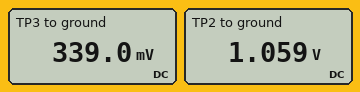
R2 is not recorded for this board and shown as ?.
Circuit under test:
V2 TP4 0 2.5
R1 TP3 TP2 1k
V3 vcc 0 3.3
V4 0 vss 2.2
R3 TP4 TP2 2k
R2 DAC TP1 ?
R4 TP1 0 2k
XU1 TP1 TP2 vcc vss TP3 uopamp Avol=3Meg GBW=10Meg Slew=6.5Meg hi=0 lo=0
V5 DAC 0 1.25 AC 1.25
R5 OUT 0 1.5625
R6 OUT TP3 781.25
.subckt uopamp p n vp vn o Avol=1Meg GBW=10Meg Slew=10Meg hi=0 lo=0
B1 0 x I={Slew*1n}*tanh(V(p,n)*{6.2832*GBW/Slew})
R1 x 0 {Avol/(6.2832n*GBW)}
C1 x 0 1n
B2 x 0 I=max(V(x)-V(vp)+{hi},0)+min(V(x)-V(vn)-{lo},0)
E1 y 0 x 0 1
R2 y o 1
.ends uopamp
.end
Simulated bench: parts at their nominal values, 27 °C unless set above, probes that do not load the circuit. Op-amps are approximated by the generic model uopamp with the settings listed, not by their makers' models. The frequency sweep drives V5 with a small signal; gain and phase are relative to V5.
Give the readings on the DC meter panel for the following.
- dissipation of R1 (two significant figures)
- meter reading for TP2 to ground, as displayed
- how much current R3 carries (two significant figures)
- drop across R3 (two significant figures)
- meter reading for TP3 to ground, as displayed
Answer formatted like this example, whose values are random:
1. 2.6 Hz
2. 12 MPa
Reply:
1. 520 µW
2. 1.059 V
3. 720 µA
4. 1.4 V
5. 339.0 mV
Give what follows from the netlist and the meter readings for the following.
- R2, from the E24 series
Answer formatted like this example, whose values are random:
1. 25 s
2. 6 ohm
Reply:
1. 360 Ω
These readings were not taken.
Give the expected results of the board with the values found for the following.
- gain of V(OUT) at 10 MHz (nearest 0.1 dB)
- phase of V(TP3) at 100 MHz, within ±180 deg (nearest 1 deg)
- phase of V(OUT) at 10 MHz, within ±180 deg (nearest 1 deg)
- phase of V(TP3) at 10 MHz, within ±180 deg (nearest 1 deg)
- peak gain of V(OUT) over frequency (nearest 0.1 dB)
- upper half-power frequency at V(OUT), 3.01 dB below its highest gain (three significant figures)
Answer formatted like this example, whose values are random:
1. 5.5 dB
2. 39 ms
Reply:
1. -57.0 dB
2. -86 deg
3. -56 deg
4. -56 deg
5. -51.9 dB
6. 6.66 MHz
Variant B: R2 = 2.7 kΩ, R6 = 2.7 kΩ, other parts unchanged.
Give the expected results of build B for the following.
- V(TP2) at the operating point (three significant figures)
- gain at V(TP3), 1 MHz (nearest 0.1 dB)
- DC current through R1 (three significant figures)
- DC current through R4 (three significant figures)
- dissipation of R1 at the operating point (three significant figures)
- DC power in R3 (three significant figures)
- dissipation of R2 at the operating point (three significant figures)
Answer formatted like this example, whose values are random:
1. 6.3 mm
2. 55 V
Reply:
1. 532 mV
2. -4.0 dB
3. 984 µA
4. 266 µA
5. 968 µW
6. 1.94 mW
7. 191 µW
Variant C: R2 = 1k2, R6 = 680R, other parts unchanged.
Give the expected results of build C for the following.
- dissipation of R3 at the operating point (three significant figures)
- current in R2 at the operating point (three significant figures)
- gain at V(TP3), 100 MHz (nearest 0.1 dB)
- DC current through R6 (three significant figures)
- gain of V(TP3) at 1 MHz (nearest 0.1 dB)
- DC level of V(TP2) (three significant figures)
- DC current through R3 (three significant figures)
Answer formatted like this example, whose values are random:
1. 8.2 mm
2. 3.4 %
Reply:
1. 1.48 mW
2. 391 µA
3. -24.1 dB
4. 115 µA
5. -0.7 dB
6. 781 mV
7. 859 µA
